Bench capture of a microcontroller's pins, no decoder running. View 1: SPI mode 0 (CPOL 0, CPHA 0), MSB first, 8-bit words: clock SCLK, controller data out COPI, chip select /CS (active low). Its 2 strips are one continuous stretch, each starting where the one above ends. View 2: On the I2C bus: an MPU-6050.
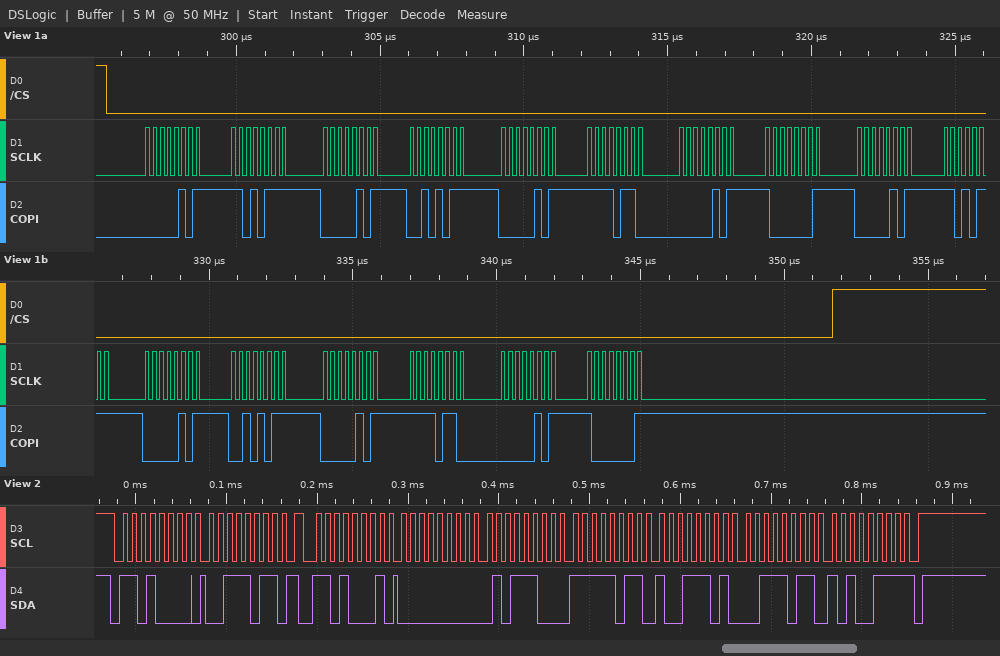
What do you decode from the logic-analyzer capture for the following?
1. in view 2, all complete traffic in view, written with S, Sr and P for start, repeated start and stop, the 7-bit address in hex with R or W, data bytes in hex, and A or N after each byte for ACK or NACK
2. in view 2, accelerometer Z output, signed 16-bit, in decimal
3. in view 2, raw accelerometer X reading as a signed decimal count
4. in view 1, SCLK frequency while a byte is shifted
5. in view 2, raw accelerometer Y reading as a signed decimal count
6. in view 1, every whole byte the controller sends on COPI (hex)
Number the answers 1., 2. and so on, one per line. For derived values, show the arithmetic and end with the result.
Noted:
1. S 68W A 3B A Sr 68R A 00 A 5C A FB A 9D A 3B A A7 N P
2. 0x3BA7 = 15271
3. 0x005C = 92
4. 4 MHz
5. 0xFB9D = -1123
6. 0x05 0xD7 0x05 0x2B 0x05 0xF6 0x05 0x81 0x05 0xD7 0x05 0x2B 0x05 0xF6 0x05 0x81
